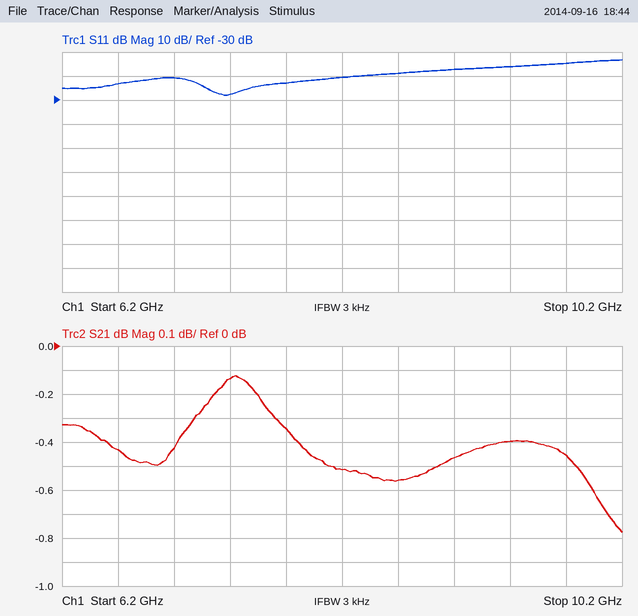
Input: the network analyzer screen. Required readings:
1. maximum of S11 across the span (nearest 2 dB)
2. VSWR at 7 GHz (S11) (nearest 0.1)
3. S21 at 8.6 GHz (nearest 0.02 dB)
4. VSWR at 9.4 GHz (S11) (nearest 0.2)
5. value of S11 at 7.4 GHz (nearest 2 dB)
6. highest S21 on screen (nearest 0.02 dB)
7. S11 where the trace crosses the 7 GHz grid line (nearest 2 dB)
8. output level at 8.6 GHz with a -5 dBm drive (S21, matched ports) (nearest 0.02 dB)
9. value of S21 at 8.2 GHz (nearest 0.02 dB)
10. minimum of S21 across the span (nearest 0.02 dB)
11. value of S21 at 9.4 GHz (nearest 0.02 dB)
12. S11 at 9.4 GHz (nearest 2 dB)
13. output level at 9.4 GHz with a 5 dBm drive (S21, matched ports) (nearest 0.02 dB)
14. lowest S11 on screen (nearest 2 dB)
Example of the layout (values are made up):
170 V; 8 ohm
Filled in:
-14 dB; 1.2; -0.56 dB; 1.4; -28 dB; -0.12 dB; -20 dB; -5.56 dBm; -0.52 dB; -0.78 dB; -0.40 dB; -16 dB; 4.60 dBm; -28 dB
